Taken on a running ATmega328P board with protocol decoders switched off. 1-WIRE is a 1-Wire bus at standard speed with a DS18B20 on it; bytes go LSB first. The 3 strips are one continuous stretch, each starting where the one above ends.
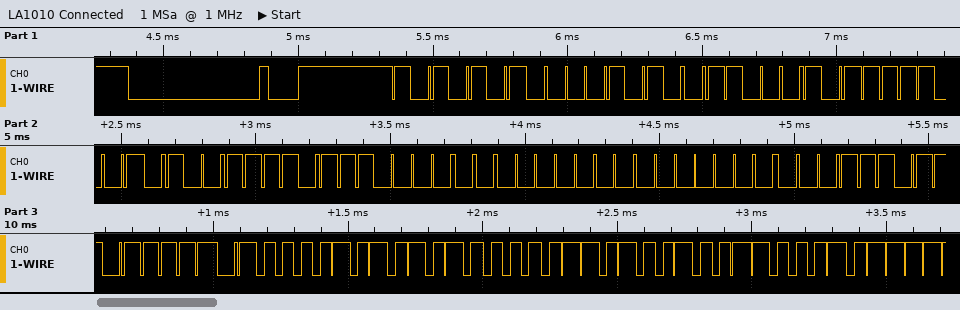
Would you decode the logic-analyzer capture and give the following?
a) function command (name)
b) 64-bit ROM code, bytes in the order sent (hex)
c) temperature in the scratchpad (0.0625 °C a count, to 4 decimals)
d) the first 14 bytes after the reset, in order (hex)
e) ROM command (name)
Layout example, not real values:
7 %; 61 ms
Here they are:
Read Scratchpad; 28 A3 4F 79 07 00 00 DC; 85.0000 °C; 55 28 A3 4F 79 07 00 00 DC BE 50 05 4B 46; Match ROM
